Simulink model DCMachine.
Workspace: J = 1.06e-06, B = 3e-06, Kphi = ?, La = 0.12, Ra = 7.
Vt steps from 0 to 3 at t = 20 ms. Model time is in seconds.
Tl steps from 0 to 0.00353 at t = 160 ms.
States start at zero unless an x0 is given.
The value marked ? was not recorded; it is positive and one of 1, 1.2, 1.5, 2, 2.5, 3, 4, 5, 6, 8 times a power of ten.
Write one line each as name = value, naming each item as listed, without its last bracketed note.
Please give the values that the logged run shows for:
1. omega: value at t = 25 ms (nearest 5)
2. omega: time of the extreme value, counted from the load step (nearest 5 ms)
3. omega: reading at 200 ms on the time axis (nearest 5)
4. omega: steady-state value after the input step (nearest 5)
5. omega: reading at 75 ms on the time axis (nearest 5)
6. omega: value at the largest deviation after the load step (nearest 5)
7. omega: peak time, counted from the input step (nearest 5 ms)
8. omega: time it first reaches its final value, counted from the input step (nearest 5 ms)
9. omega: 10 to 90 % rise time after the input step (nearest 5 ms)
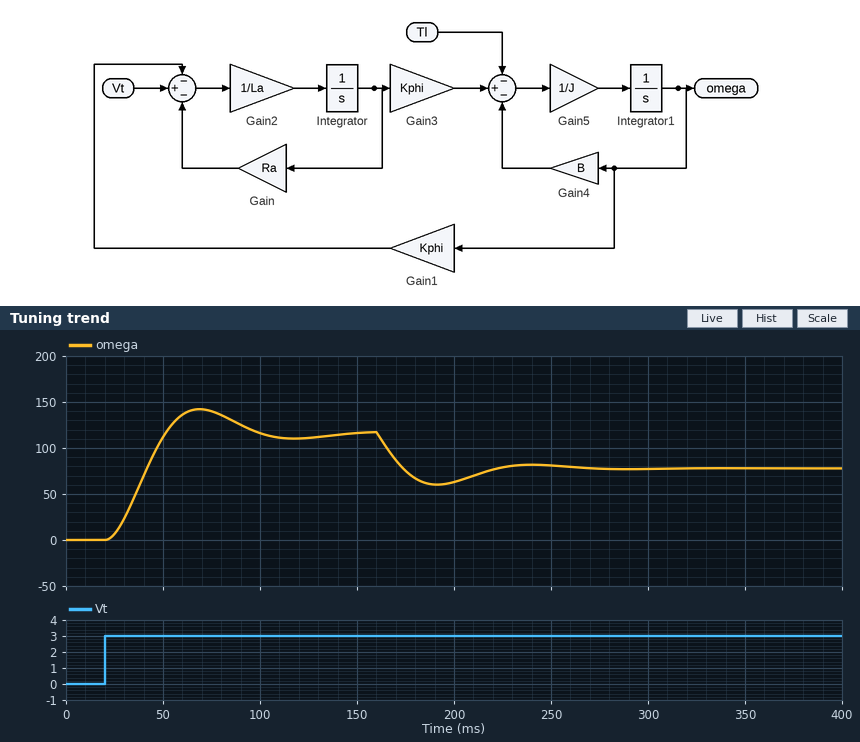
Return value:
omega: value at t = 25 ms = 5
omega: time of the extreme value, counted from the load step = 30 ms
omega: reading at 200 ms on the time axis = 65
omega: steady-state value after the input step = 115
omega: reading at 75 ms on the time axis = 140
omega: value at the largest deviation after the load step = 60
omega: peak time, counted from the input step = 50 ms
omega: time it first reaches its final value, counted from the input step = 30 ms
omega: 10 to 90 % rise time after the input step = 20 ms
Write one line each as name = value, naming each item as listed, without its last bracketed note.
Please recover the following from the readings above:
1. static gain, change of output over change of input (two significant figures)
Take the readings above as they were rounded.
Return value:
static gain, change of output over change of input = 38
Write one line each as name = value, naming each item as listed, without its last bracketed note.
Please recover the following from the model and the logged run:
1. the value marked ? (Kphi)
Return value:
the value marked ? = 0.025
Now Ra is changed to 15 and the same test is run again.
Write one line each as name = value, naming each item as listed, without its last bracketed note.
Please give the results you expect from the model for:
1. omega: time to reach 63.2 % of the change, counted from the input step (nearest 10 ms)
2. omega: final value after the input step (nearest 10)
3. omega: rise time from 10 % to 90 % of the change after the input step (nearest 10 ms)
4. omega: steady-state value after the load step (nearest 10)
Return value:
omega: time to reach 63.2 % of the change, counted from the input step = 30 ms
omega: final value after the input step = 110
omega: rise time from 10 % to 90 % of the change after the input step = 40 ms
omega: steady-state value after the load step = 30
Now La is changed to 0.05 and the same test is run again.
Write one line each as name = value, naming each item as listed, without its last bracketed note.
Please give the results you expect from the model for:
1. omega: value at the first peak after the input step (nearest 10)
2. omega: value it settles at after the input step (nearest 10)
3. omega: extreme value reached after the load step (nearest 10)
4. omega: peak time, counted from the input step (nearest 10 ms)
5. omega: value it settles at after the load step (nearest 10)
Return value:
omega: value at the first peak after the input step = 120
omega: value it settles at after the input step = 120
omega: extreme value reached after the load step = 70
omega: peak time, counted from the input step = 40 ms
omega: value it settles at after the load step = 80
